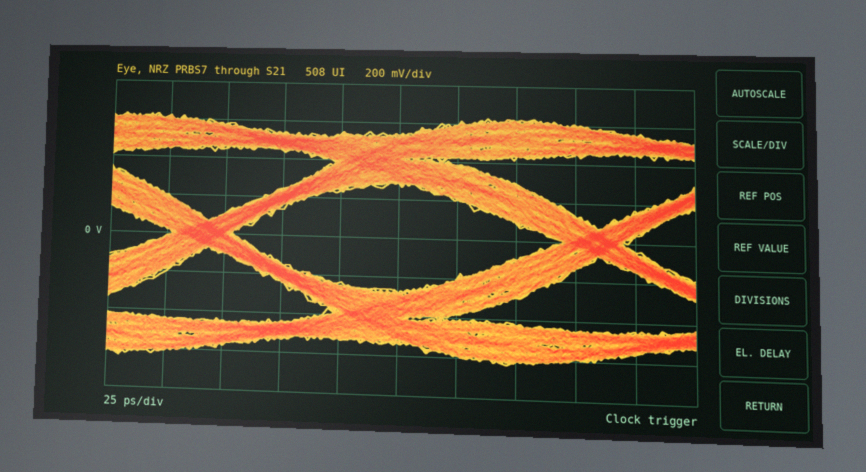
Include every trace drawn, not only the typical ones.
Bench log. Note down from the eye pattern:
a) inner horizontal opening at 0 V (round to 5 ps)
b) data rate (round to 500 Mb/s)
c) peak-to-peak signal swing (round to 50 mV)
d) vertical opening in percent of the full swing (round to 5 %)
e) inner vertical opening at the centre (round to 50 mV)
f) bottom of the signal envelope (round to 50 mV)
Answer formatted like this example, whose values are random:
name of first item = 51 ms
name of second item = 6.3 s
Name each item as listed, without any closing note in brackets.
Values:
inner horizontal opening at 0 V = 140 ps
data rate = 6.0 Gb/s
peak-to-peak signal swing = 1.25 V
vertical opening in percent of the full swing = 45 %
inner vertical opening at the centre = 550 mV
bottom of the signal envelope = -650 mV
